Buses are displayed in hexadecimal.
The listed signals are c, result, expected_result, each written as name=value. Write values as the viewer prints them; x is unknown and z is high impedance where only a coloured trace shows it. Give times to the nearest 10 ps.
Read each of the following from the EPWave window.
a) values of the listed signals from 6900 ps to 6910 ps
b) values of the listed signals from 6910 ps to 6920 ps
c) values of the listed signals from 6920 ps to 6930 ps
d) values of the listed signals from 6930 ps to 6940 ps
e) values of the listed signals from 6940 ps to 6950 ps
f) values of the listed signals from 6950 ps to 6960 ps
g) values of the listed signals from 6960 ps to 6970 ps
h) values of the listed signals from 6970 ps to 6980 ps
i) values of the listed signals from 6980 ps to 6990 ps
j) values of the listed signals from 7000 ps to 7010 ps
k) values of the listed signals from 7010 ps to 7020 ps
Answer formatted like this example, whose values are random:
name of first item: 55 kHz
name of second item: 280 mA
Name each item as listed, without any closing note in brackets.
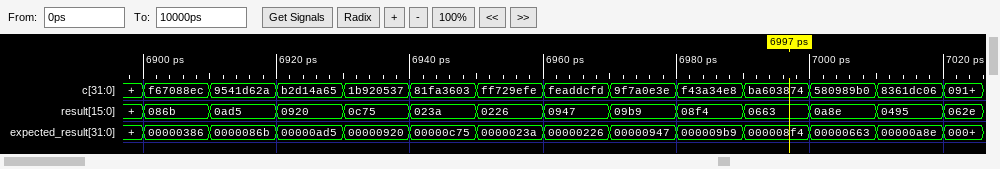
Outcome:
values of the listed signals from 6900 ps to 6910 ps: c=f67088ec, result=086b, expected_result=00000386
values of the listed signals from 6910 ps to 6920 ps: c=9541d62a, result=0ad5, expected_result=0000086b
values of the listed signals from 6920 ps to 6930 ps: c=b2d14a65, result=0920, expected_result=00000ad5
values of the listed signals from 6930 ps to 6940 ps: c=1b920537, result=0c75, expected_result=00000920
values of the listed signals from 6940 ps to 6950 ps: c=81fa3603, result=023a, expected_result=00000c75
values of the listed signals from 6950 ps to 6960 ps: c=ff729efe, result=0226, expected_result=0000023a
values of the listed signals from 6960 ps to 6970 ps: c=feaddcfd, result=0947, expected_result=00000226
values of the listed signals from 6970 ps to 6980 ps: c=9f7a0e3e, result=09b9, expected_result=00000947
values of the listed signals from 6980 ps to 6990 ps: c=f43a34e8, result=08f4, expected_result=000009b9
values of the listed signals from 7000 ps to 7010 ps: c=580989b0, result=0a8e, expected_result=00000663
values of the listed signals from 7010 ps to 7020 ps: c=8361dc06, result=0495, expected_result=00000a8e
